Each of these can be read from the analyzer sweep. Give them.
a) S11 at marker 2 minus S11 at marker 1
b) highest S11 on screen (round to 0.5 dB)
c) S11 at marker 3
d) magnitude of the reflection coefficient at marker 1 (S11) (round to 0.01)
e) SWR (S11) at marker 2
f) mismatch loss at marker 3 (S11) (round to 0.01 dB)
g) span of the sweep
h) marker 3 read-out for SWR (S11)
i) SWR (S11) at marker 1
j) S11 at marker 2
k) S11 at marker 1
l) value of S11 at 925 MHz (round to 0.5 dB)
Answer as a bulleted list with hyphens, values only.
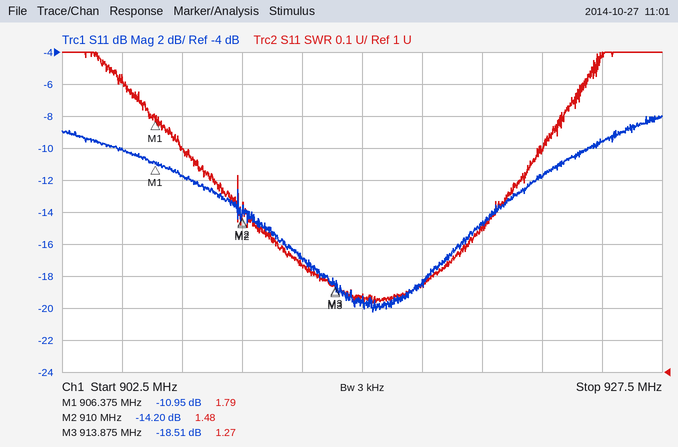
- -3.25 dB
- -8.0 dB
- -18.51 dB
- 0.28
- 1.48
- 0.06 dB
- 25 MHz
- 1.27
- 1.79
- -14.20 dB
- -10.95 dB
- -9.5 dB
